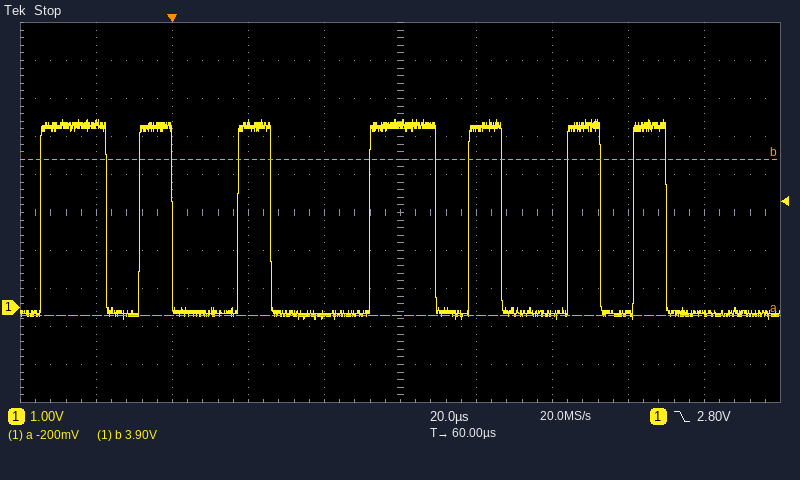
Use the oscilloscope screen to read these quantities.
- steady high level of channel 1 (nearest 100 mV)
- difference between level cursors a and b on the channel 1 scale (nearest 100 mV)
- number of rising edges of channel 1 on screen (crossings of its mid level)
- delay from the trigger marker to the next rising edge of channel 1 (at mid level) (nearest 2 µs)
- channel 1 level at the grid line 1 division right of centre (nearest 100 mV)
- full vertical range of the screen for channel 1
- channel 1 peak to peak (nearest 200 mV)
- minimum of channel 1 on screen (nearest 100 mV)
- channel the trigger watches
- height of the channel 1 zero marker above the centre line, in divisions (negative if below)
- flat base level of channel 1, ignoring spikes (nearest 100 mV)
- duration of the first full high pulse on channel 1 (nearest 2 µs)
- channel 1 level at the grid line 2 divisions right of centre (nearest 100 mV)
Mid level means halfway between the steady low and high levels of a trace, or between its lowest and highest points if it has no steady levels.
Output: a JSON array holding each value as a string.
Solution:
["4.8 V", "4.1 V", "7", "18 µs", "4.7 V", "10 V", "5.2 V", "-300 mV", "channel 1", "-2.5 div", "-200 mV", "18 µs", "-200 mV"]
